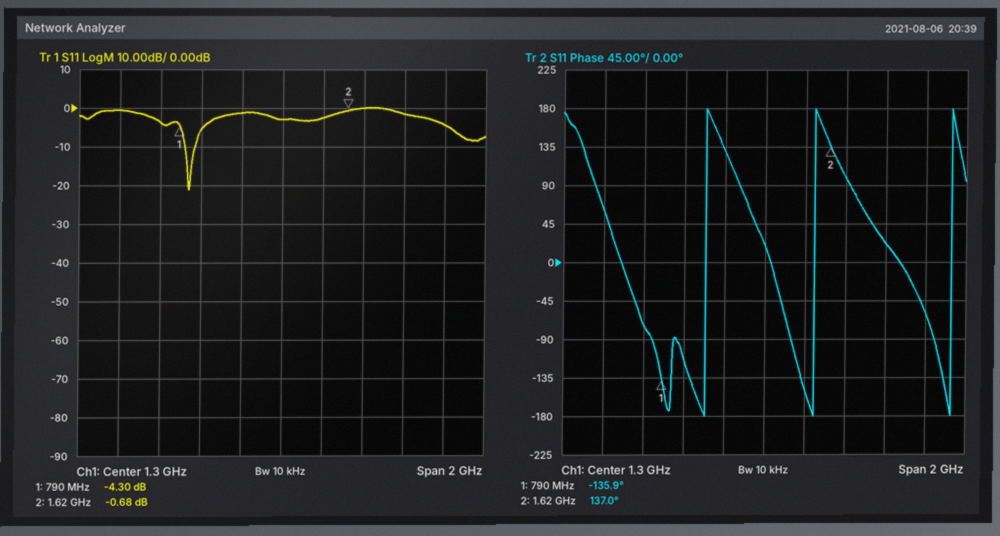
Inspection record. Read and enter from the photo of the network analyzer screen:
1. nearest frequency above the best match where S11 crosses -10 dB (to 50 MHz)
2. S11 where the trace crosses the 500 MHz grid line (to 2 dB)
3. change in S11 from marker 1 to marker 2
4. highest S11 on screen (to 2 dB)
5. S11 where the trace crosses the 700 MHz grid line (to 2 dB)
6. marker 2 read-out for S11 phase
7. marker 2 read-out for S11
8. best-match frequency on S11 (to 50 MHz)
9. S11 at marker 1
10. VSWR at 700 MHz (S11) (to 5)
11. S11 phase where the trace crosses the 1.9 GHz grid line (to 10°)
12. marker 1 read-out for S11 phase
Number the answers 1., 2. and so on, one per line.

1. 850 MHz
2. 0 dB
3. 3.62 dB
4. 0 dB
5. -4 dB
6. 137.0°
7. -0.68 dB
8. 850 MHz
9. -4.30 dB
10. 5
11. 20°
12. -135.9°
